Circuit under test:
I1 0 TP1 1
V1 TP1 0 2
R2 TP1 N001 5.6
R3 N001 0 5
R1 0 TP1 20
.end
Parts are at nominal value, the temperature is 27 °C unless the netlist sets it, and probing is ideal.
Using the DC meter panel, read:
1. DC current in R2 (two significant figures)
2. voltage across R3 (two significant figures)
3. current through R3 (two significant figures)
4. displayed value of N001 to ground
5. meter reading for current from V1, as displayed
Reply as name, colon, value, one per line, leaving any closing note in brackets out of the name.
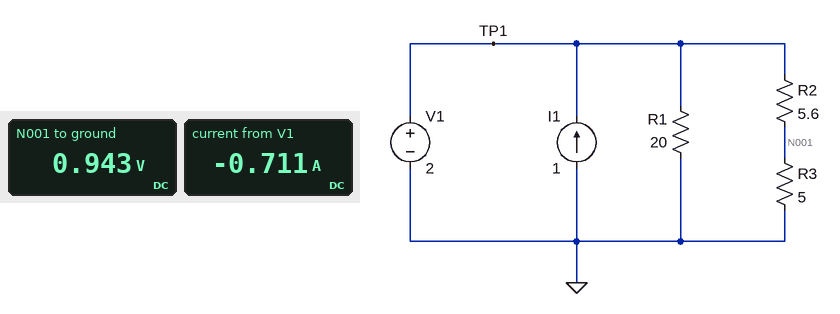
DC current in R2: 190 mA
voltage across R3: 940 mV
current through R3: 190 mA
displayed value of N001 to ground: 0.943 V
meter reading for current from V1, as displayed: -0.711 A
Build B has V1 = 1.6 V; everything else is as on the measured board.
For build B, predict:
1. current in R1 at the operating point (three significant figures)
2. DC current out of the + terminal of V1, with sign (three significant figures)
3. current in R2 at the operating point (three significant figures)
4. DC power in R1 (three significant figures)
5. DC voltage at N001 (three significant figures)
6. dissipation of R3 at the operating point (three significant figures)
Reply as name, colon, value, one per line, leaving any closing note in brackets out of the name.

current in R1 at the operating point: 80.0 mA
DC current out of the + terminal of V1, with sign: -769 mA
current in R2 at the operating point: 151 mA
DC power in R1: 128 mW
DC voltage at N001: 755 mV
dissipation of R3 at the operating point: 114 mW
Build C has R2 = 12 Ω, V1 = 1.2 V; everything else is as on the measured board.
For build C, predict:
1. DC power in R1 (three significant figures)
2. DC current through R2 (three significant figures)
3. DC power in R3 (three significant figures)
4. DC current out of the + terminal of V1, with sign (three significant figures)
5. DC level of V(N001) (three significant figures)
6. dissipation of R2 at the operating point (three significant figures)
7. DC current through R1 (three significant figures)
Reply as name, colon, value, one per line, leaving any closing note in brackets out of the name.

DC power in R1: 72.0 mW
DC current through R2: 70.6 mA
DC power in R3: 24.9 mW
DC current out of the + terminal of V1, with sign: -869 mA
DC level of V(N001): 353 mV
dissipation of R2 at the operating point: 59.8 mW
DC current through R1: 60.0 mA
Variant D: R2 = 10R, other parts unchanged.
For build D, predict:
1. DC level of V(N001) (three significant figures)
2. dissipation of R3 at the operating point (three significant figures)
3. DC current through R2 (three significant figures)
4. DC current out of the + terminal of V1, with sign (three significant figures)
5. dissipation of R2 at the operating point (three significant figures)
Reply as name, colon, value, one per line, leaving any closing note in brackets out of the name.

DC level of V(N001): 667 mV
dissipation of R3 at the operating point: 88.9 mW
DC current through R2: 133 mA
DC current out of the + terminal of V1, with sign: -767 mA
dissipation of R2 at the operating point: 178 mW
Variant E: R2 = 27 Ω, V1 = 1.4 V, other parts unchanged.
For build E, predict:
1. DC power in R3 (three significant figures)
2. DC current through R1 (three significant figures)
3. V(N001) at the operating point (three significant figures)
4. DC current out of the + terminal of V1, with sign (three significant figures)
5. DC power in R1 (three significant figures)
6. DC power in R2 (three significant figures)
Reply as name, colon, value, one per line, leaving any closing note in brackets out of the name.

DC power in R3: 9.57 mW
DC current through R1: 70.0 mA
V(N001) at the operating point: 219 mV
DC current out of the + terminal of V1, with sign: -886 mA
DC power in R1: 98.0 mW
DC power in R2: 51.7 mW
